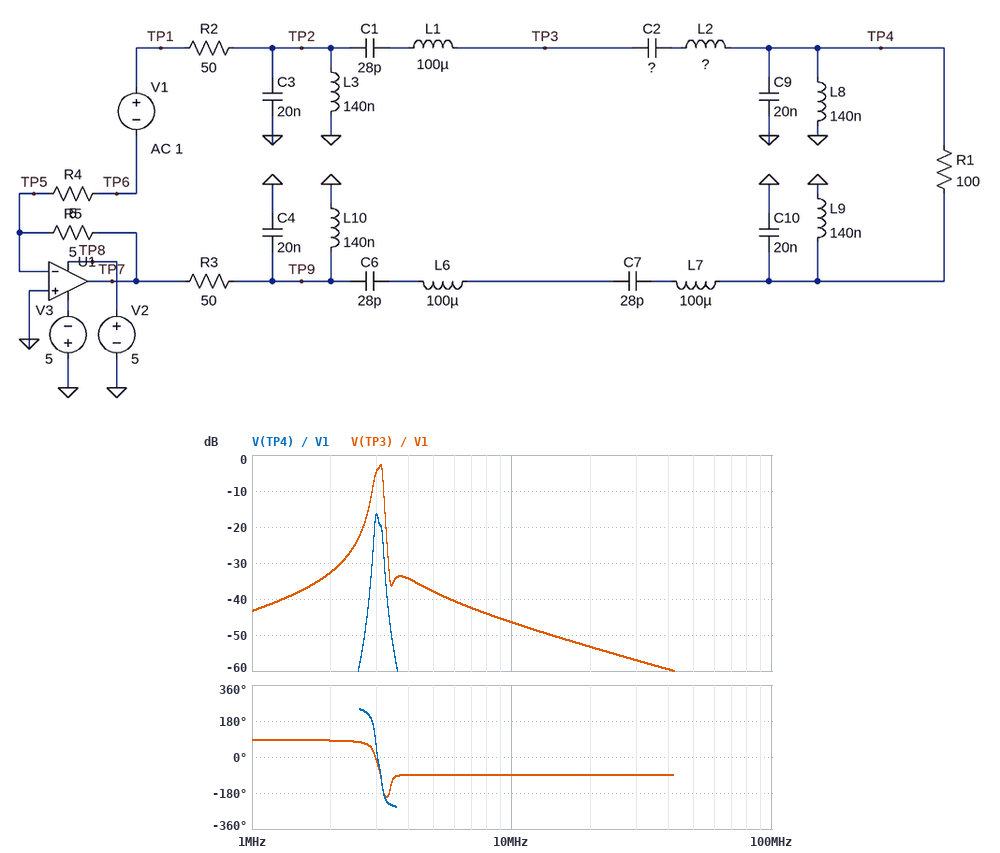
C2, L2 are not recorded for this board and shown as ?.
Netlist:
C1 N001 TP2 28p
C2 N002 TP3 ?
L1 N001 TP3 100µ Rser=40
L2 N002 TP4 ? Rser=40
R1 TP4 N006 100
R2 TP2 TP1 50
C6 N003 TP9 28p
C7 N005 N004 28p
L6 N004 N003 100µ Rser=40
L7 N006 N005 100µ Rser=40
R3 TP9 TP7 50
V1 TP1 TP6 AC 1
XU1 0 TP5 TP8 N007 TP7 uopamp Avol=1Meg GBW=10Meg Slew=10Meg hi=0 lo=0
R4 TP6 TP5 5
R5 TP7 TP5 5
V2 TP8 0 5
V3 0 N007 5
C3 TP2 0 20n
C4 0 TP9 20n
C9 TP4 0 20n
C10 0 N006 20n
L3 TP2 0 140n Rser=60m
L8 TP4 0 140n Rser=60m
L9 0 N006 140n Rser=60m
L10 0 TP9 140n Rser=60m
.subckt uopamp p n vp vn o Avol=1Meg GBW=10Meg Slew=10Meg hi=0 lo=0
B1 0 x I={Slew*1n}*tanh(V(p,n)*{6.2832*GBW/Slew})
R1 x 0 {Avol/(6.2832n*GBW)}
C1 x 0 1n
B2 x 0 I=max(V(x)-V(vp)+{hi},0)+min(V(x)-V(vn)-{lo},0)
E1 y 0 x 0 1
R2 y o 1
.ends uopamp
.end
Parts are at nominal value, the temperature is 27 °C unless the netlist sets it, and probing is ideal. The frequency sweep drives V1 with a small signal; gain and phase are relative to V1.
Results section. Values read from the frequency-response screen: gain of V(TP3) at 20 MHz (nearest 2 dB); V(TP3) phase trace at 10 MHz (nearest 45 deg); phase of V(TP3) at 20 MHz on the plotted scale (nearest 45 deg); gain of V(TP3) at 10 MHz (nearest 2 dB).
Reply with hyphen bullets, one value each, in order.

- -54 dB
- -90 deg
- -90 deg
- -46 dB
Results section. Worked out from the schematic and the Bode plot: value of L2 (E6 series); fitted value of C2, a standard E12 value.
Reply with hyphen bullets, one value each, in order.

- 47 µH
- 47 pF
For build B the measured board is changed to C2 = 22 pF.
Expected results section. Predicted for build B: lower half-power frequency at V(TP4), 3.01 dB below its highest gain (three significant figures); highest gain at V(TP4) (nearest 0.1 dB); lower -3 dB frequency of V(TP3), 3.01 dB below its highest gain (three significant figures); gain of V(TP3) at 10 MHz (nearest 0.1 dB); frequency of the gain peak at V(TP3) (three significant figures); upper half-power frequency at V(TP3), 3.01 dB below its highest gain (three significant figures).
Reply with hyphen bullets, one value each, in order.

- 2.96 MHz
- -30.7 dB
- 3.69 MHz
- -47.5 dB
- 3.74 MHz
- 3.78 MHz
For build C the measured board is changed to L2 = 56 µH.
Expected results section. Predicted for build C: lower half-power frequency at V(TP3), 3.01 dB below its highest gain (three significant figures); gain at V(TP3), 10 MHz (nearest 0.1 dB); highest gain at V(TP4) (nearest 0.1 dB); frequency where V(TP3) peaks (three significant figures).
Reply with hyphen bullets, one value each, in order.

- 2.95 MHz
- -45.4 dB
- -12.6 dB
- 3.03 MHz
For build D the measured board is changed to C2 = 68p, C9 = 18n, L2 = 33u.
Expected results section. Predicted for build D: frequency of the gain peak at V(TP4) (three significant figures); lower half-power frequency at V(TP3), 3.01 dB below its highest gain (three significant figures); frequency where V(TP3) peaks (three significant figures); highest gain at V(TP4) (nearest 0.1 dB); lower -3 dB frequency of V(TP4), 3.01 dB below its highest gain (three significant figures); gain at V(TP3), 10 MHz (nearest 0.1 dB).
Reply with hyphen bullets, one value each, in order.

- 3.09 MHz
- 2.94 MHz
- 3.03 MHz
- -14.7 dB
- 3.04 MHz
- -48.7 dB
